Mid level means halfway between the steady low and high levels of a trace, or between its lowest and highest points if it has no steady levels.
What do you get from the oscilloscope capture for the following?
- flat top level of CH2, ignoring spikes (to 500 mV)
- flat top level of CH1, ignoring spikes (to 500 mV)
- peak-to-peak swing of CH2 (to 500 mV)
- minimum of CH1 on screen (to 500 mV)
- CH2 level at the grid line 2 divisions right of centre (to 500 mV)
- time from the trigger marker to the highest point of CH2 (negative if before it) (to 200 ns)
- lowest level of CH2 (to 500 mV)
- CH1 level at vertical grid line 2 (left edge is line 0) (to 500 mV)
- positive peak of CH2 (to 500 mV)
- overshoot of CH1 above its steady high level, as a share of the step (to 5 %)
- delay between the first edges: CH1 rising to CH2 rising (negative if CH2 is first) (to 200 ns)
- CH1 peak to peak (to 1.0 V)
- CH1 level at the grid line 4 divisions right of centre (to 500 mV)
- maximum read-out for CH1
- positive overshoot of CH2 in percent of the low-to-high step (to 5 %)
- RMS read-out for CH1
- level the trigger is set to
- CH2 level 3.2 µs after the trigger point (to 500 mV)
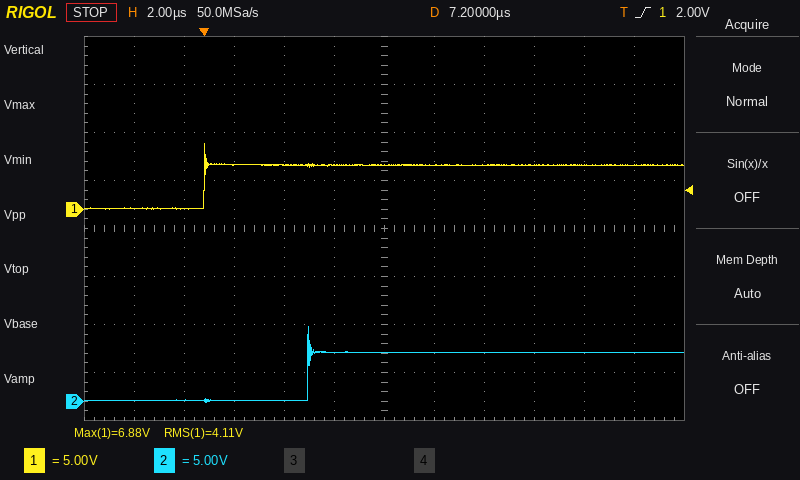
5.0 V
4.5 V
8.0 V
0.0 V
5.0 V
+4.2 µs
0.0 V
0.0 V
8.0 V
50 %
+4.2 µs
7.0 V
4.5 V
6.88 V
55 %
4.11 V
2.00 V
0.0 V
